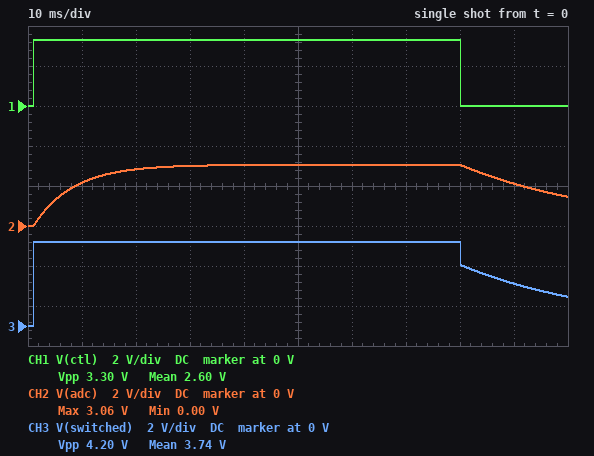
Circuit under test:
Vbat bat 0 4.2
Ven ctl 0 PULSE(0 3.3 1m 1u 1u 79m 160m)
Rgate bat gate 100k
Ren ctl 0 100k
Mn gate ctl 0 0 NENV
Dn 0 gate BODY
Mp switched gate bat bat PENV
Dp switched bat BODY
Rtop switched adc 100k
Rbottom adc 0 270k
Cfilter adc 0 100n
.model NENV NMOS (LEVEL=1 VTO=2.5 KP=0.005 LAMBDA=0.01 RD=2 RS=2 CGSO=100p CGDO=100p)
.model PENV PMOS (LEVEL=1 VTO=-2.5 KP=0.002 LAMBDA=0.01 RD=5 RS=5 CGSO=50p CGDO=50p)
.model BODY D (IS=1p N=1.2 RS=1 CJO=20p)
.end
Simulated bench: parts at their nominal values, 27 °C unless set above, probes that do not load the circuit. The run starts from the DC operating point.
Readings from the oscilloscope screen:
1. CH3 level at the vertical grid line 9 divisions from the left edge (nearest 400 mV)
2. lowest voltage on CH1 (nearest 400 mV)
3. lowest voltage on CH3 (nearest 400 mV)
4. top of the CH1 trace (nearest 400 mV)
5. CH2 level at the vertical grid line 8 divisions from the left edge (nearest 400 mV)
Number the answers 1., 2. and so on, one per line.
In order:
1. 2.0 V
2. 0 V
3. 0 V
4. 3.2 V
5. 3.2 V
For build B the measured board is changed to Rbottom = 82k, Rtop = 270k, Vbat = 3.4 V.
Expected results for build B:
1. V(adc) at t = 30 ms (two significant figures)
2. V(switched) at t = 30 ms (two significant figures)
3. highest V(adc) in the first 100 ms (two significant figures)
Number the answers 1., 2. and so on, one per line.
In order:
1. 780 mV
2. 3.4 V
3. 790 mV
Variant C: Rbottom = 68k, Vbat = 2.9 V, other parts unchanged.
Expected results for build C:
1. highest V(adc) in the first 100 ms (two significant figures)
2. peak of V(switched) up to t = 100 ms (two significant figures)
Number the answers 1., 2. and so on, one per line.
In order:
1. 1.2 V
2. 2.9 V
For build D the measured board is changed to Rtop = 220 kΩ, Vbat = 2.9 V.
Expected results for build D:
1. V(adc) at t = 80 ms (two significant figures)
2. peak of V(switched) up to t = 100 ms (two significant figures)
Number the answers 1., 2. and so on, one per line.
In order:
1. 1.6 V
2. 2.9 V
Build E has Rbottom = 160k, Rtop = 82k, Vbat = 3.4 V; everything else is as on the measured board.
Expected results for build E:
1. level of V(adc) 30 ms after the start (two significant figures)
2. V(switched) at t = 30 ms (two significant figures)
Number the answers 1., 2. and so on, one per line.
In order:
1. 2.2 V
2. 3.4 V
